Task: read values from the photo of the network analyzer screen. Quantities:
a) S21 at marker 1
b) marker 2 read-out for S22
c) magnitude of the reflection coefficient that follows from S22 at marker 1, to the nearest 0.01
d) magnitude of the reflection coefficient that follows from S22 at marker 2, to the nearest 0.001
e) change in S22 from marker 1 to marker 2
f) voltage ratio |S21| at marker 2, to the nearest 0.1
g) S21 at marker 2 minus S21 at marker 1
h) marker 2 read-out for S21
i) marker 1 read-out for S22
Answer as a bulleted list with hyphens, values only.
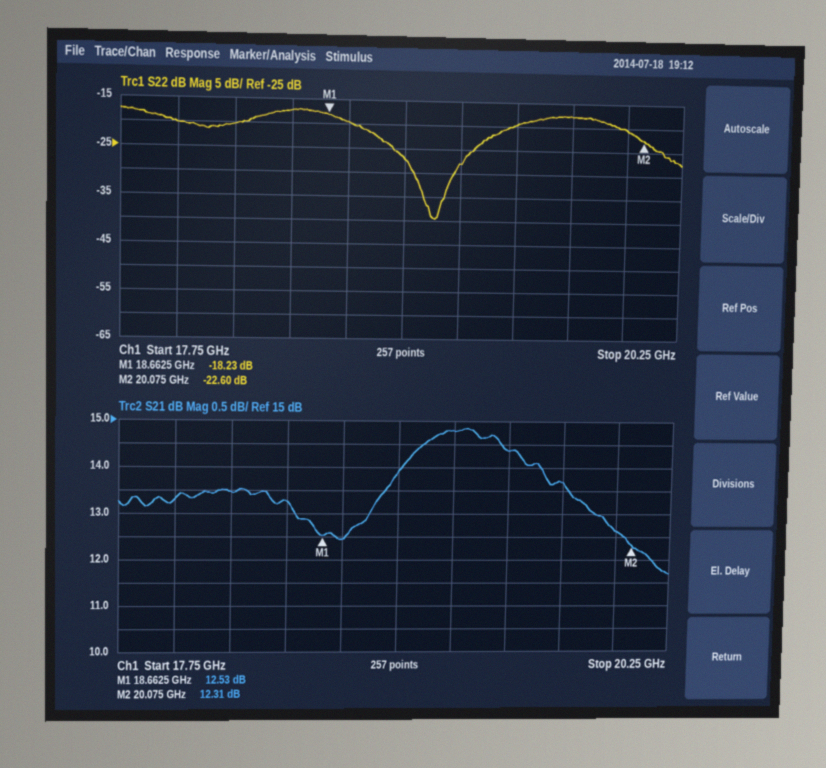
- 12.53 dB
- -22.60 dB
- 0.12
- 0.074
- -4.37 dB
- 4.1
- -0.22 dB
- 12.31 dB
- -18.23 dB
